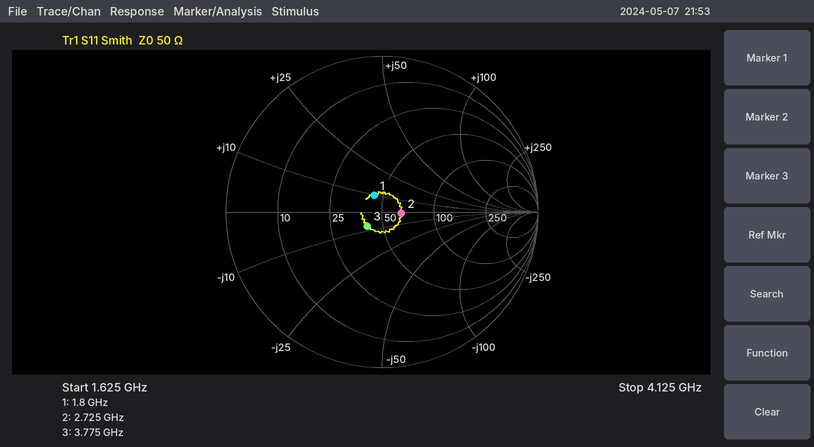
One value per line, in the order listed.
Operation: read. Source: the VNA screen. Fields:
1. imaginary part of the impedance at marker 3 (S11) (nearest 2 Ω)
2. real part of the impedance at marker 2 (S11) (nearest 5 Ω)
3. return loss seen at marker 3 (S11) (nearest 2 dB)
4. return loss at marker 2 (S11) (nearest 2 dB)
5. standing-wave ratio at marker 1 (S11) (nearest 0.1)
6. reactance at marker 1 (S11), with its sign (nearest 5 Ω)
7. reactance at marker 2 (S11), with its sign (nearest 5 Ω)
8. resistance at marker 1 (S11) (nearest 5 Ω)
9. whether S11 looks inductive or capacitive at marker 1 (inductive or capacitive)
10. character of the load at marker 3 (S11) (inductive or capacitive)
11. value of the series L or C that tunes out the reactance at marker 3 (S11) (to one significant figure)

-8 Ω
65 Ω
18 dB
18 dB
1.3
+10 Ω
0 Ω
45 Ω
inductive
capacitive
300 pH
